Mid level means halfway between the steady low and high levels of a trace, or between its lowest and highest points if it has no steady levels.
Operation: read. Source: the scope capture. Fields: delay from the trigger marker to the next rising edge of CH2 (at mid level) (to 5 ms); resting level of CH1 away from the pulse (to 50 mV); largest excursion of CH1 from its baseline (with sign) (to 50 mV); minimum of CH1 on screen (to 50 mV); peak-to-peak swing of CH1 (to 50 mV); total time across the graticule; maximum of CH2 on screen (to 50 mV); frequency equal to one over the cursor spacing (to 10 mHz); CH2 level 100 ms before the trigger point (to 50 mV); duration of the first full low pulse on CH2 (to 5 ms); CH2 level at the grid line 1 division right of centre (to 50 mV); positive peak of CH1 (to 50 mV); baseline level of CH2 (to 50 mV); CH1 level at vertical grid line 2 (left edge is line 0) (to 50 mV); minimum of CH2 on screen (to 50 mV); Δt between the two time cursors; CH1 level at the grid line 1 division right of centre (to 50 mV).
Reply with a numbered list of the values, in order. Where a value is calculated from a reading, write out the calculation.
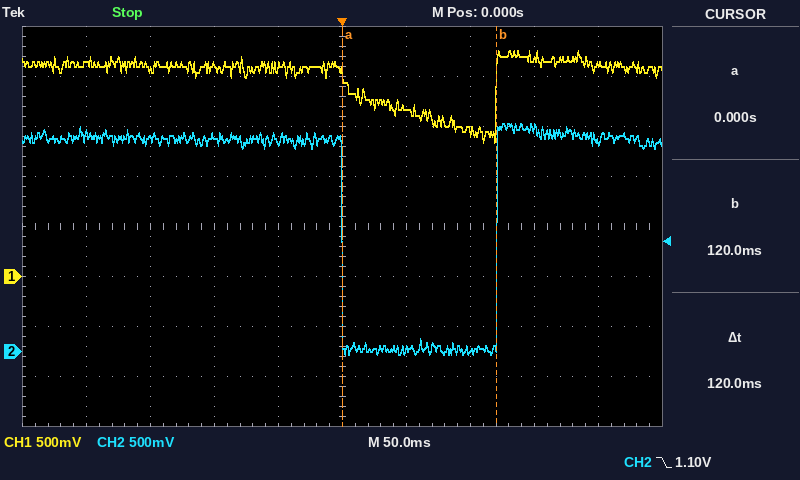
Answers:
1. 120 ms
2. 2.10 V
3. 1.35 V − (2.10 V) = -750 mV
4. 1.35 V
5. 2.25 V − (1.35 V) = 900 mV
6. 500 ms
7. 2.30 V
8. 1 / 120 ms ≈ 8.33 Hz
9. 2.15 V
10. 120 ms
11. 0 mV
12. 2.25 V
13. 2.15 V
14. 2.05 V
15. -50 mV
16. 120 ms
17. 1.70 V
